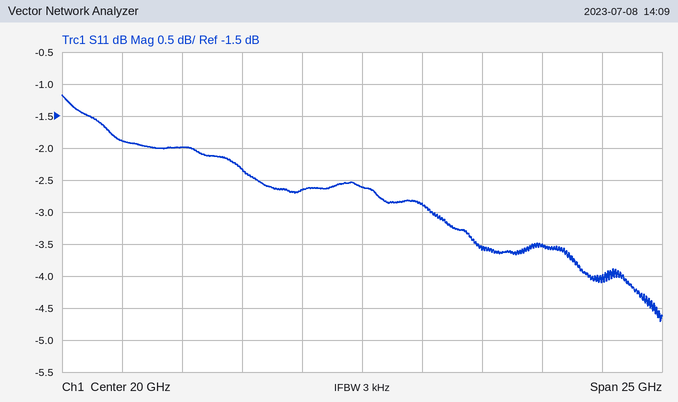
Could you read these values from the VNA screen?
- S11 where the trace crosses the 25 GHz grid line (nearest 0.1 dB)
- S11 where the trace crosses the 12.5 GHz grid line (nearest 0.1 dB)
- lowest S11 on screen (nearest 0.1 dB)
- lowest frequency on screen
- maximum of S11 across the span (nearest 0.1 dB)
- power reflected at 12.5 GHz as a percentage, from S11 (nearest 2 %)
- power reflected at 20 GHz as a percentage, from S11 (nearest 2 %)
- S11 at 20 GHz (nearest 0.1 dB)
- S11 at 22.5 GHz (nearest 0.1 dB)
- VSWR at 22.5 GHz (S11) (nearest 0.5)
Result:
-3.6 dB
-2.0 dB
-4.7 dB
7.5 GHz
-1.2 dB
64 %
54 %
-2.6 dB
-2.9 dB
6.0
